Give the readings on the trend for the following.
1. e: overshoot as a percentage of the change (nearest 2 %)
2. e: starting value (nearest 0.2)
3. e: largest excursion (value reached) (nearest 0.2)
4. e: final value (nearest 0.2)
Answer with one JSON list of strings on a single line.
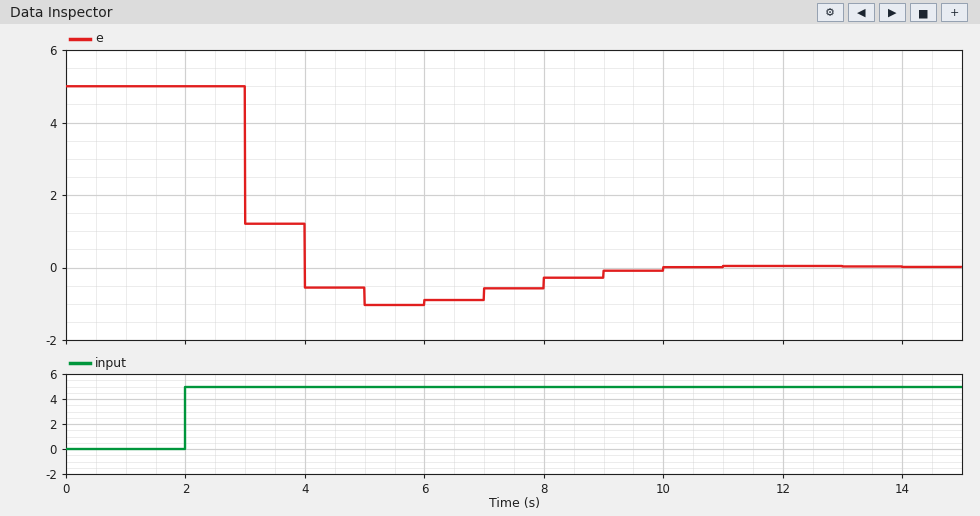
["20 %", "5.0", "-1.0", "0.0"]
